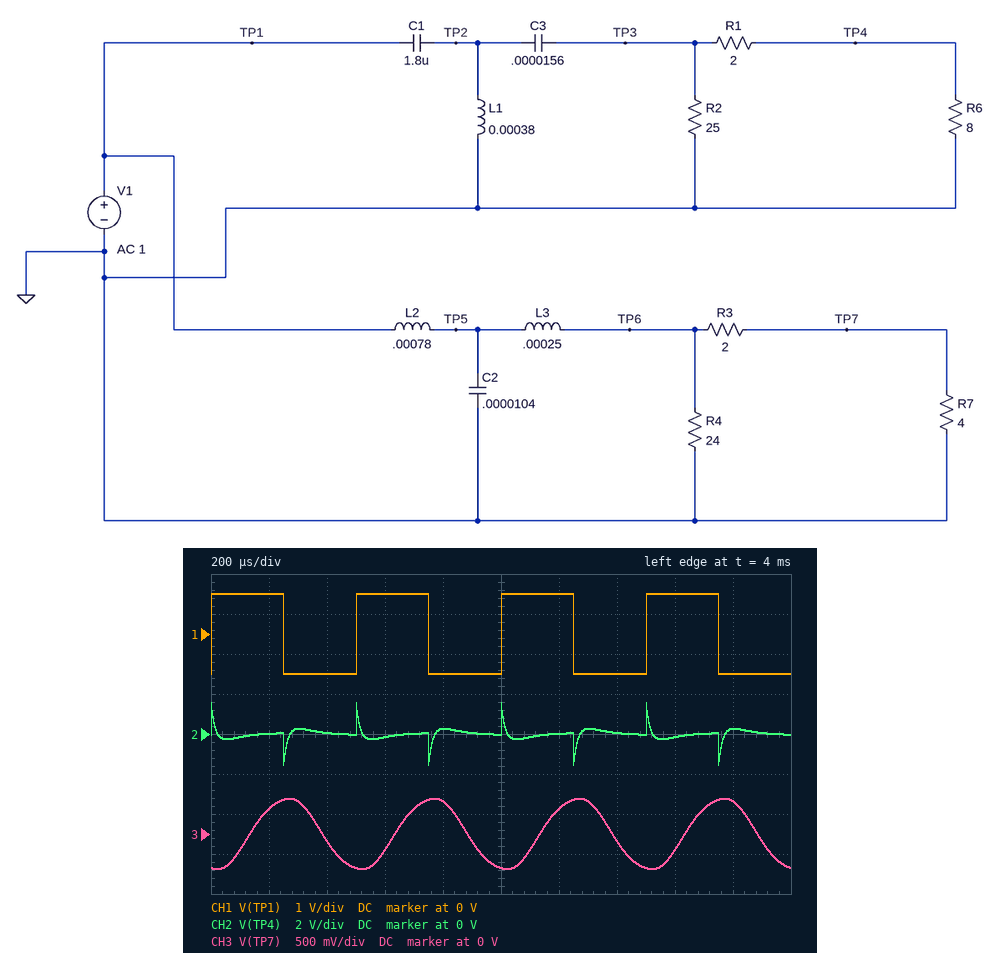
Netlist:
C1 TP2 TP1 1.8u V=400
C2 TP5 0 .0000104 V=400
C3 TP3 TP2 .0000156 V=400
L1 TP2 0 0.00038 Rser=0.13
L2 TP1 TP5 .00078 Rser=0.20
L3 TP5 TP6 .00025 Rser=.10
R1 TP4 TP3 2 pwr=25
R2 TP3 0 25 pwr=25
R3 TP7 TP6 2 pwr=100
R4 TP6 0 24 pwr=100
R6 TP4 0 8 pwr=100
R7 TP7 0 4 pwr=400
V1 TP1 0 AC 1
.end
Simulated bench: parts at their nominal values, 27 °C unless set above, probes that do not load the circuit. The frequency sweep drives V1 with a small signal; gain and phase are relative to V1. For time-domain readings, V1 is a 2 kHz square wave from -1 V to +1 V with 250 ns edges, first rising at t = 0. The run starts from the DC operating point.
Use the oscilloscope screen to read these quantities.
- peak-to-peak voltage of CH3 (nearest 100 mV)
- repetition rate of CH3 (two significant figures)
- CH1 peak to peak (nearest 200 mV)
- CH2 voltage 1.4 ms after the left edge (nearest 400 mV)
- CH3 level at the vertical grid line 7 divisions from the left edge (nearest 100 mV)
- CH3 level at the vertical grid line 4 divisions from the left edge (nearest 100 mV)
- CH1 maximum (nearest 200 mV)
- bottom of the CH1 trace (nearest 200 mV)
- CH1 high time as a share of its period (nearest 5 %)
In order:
900 mV
2.0 kHz
2.0 V
0 V
-100 mV
400 mV
1.0 V
-1.0 V
50 %
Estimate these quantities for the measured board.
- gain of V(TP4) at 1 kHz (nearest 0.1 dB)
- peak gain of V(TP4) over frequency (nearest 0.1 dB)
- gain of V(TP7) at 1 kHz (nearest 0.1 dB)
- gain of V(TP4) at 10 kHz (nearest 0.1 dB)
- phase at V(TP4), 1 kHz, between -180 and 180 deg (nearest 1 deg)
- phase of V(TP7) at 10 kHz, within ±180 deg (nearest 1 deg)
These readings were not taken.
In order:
-36.5 dB
-1.9 dB
-6.8 dB
-5.3 dB
-136 deg
109 deg
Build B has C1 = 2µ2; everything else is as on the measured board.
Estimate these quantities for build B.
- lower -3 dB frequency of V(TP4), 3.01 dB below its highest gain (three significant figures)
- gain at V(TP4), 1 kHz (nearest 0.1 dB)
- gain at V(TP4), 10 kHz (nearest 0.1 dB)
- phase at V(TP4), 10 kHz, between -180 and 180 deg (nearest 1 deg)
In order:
8.52 kHz
-34.7 dB
-4.3 dB
58 deg
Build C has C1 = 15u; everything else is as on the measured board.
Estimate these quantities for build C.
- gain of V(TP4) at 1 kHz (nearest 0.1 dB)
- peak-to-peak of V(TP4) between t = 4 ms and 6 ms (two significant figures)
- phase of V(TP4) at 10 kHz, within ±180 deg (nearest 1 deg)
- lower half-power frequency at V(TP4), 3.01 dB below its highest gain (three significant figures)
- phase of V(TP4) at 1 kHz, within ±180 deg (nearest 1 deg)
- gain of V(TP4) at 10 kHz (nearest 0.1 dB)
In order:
-15.8 dB
5.1 V
17 deg
1.53 kHz
-140 deg
-1.9 dB
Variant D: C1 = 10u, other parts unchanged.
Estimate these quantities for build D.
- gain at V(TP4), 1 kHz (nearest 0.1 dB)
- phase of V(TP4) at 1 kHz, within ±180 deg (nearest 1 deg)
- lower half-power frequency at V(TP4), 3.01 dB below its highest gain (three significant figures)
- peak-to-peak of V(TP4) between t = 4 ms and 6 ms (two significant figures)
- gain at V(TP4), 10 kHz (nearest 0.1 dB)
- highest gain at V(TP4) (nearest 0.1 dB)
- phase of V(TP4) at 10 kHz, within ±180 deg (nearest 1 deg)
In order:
-20.3 dB
-138 deg
1.77 kHz
3.9 V
-1.9 dB
-0.8 dB
21 deg
